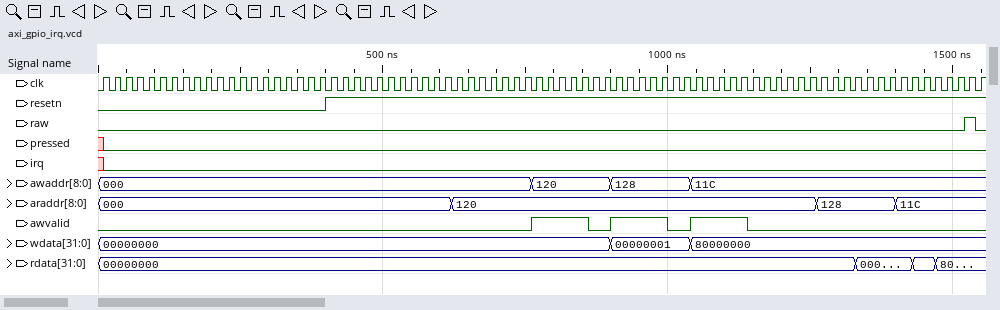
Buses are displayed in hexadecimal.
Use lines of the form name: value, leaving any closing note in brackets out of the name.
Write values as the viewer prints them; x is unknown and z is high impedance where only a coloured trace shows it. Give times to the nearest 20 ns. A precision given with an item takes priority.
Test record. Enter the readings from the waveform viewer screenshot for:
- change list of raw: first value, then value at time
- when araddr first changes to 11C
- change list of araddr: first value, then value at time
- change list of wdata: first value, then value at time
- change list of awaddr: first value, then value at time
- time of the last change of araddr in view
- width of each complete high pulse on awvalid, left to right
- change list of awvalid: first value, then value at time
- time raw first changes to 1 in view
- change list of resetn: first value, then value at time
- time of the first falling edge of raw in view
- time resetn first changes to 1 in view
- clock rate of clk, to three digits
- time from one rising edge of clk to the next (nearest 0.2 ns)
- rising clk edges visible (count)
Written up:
change list of raw: first value, then value at time: 0, 1 at 1520 ns, 0 at 1540 ns
when araddr first changes to 11C: 1400 ns
change list of araddr: first value, then value at time: 000, 120 at 620 ns, 128 at 1260 ns, 11C at 1400 ns
change list of wdata: first value, then value at time: 00000000, 00000001 at 900 ns, 80000000 at 1040 ns
change list of awaddr: first value, then value at time: 000, 120 at 760 ns, 128 at 900 ns, 11C at 1040 ns
time of the last change of araddr in view: 1400 ns
width of each complete high pulse on awvalid, left to right: 100 ns, 100 ns, 100 ns
change list of awvalid: first value, then value at time: 0, 1 at 760 ns, 0 at 860 ns, 1 at 900 ns, 0 at 1000 ns, 1 at 1040 ns, 0 at 1140 ns
time raw first changes to 1 in view: 1520 ns
change list of resetn: first value, then value at time: 0, 1 at 400 ns
time of the first falling edge of raw in view: 1540 ns
time resetn first changes to 1 in view: 400 ns
clock rate of clk, to three digits: 50.0 MHz
time from one rising edge of clk to the next: 20 ns
rising clk edges visible: 78
